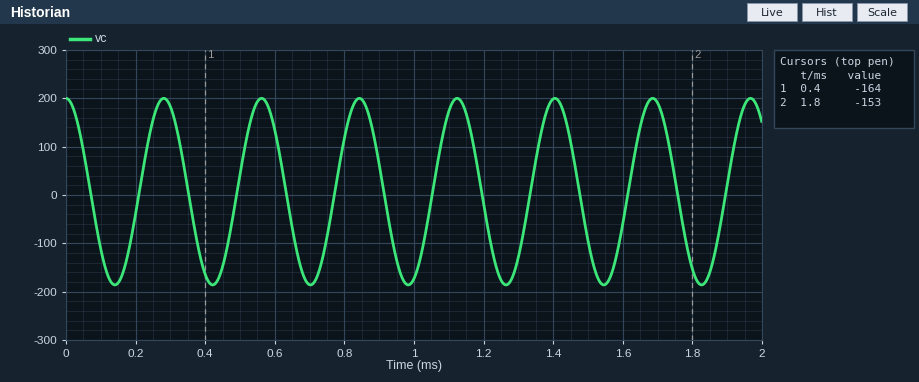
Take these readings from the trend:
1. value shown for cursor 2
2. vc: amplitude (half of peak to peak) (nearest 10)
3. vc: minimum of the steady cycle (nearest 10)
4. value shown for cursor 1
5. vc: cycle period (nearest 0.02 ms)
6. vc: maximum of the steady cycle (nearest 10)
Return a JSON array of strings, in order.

["-153", "190", "-190", "-164", "0.28 ms", "200"]
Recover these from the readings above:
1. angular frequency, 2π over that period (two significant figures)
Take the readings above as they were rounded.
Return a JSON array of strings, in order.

["22 rad/ms"]
